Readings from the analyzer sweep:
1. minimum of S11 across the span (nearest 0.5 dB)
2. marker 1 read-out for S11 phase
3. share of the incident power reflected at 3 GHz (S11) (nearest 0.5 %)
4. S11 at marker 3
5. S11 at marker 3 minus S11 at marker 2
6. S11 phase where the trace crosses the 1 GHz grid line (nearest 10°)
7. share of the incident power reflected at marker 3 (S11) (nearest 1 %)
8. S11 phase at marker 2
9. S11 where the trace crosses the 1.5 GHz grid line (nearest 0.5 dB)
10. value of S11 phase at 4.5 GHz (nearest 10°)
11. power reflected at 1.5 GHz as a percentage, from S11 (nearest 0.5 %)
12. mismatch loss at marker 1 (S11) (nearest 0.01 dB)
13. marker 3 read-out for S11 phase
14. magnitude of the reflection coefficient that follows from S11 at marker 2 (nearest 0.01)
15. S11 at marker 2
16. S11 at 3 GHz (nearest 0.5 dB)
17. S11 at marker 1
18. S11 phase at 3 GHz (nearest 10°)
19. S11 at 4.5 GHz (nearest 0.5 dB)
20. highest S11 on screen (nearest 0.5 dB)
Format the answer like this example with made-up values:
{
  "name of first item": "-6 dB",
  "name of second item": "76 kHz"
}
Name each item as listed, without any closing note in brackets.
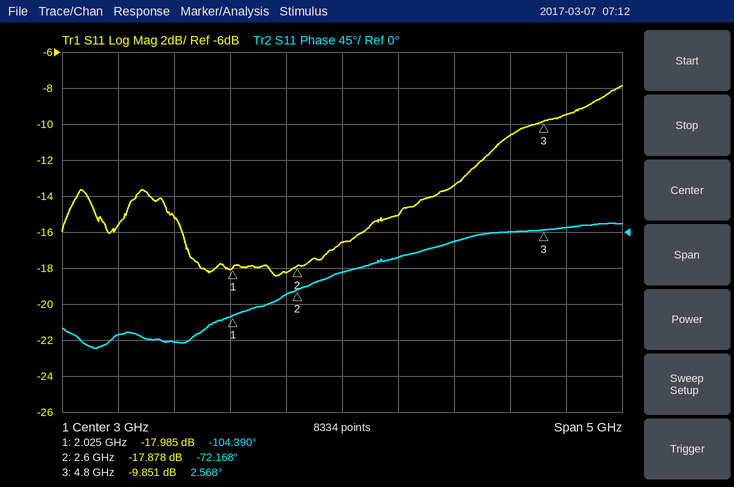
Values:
{
  "minimum of S11 across the span": "-18.5 dB",
  "marker 1 read-out for S11 phase": "-104.390°",
  "share of the incident power reflected at 3 GHz (S11)": "2.0 %",
  "S11 at marker 3": "-9.851 dB",
  "S11 at marker 3 minus S11 at marker 2": "8.027 dB",
  "S11 phase where the trace crosses the 1 GHz grid line": "-130°",
  "share of the incident power reflected at marker 3 (S11)": "10 %",
  "S11 phase at marker 2": "-72.168°",
  "S11 where the trace crosses the 1.5 GHz grid line": "-15.0 dB",
  "value of S11 phase at 4.5 GHz": "0°",
  "power reflected at 1.5 GHz as a percentage, from S11": "3.0 %",
  "mismatch loss at marker 1 (S11)": "0.07 dB",
  "marker 3 read-out for S11 phase": "2.568°",
  "magnitude of the reflection coefficient that follows from S11 at marker 2": "0.13",
  "S11 at marker 2": "-17.878 dB",
  "S11 at 3 GHz": "-16.5 dB",
  "S11 at marker 1": "-17.985 dB",
  "S11 phase at 3 GHz": "-50°",
  "S11 at 4.5 GHz": "-10.5 dB",
  "highest S11 on screen": "-8.0 dB"
}
